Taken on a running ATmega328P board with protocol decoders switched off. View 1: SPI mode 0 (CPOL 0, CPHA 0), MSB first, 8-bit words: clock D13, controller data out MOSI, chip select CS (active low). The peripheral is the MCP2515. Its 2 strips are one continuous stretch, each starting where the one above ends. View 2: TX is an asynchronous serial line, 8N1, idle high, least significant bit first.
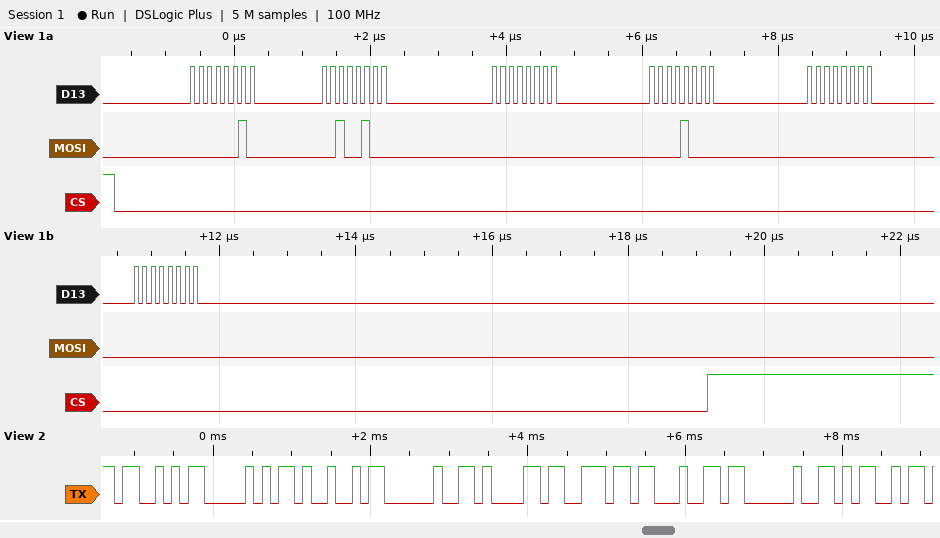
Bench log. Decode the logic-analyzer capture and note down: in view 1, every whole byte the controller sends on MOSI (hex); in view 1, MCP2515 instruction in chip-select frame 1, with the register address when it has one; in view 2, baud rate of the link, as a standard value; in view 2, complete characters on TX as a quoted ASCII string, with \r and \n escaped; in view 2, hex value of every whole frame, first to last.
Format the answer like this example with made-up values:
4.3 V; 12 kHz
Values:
02 24 00 08 00 00; WRITE 0x24; 9600 baud; "SPI and M"; 53 50 49 20 61 6E 64 20 4D
